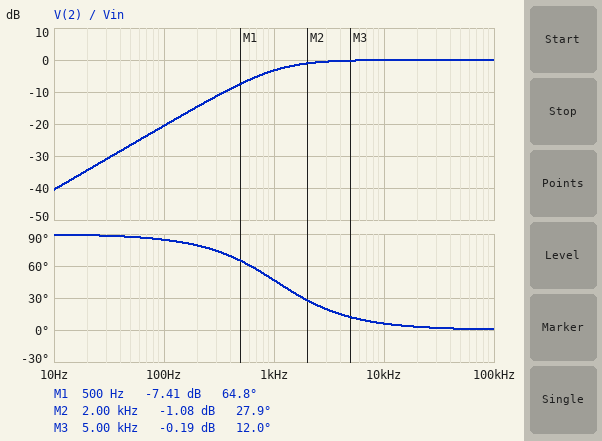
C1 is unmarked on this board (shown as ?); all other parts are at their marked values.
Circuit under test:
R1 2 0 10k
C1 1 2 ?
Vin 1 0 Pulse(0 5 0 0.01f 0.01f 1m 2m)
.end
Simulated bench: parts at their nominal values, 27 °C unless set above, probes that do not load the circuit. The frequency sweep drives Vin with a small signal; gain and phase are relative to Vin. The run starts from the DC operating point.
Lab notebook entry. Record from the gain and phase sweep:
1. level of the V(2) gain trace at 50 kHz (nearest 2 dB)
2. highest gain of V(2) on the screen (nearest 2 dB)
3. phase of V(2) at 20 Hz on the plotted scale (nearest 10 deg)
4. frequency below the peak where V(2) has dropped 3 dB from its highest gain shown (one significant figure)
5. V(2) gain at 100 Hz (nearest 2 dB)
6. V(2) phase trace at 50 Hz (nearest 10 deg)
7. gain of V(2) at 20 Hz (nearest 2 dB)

0 dB
0 dB
90 deg
1 kHz
-20 dB
90 deg
-34 dB
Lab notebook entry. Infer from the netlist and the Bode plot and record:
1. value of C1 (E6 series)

15 nF
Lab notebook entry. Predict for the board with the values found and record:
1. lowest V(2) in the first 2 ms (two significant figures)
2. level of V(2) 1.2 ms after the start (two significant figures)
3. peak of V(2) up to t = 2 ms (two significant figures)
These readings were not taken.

-5.0 V
-1.3 V
5.0 V
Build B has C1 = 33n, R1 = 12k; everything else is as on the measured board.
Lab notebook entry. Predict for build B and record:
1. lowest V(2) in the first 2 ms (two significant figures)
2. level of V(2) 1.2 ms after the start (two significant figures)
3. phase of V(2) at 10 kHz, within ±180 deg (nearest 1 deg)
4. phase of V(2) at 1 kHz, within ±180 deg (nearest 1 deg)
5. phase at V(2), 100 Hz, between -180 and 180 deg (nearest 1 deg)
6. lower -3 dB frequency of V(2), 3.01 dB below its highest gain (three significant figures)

-4.6 V
-2.8 V
2 deg
22 deg
76 deg
402 Hz
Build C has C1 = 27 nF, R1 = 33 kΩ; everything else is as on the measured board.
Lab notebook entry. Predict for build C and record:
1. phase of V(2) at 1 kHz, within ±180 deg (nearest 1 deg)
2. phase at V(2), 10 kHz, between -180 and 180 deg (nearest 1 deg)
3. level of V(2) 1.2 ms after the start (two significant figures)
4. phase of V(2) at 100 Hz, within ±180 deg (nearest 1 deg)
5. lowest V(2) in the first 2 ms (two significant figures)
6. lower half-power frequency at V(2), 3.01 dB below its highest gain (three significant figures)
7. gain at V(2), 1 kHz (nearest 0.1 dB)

10 deg
1 deg
-2.7 V
61 deg
-3.4 V
179 Hz
-0.1 dB
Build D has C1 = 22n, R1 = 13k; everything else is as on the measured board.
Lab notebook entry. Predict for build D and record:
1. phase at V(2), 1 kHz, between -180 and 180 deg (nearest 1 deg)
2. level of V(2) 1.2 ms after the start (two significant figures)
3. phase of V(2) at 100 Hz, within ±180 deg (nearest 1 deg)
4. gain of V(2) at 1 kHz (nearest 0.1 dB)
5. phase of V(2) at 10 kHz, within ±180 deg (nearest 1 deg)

29 deg
-2.4 V
80 deg
-1.2 dB
3 deg
